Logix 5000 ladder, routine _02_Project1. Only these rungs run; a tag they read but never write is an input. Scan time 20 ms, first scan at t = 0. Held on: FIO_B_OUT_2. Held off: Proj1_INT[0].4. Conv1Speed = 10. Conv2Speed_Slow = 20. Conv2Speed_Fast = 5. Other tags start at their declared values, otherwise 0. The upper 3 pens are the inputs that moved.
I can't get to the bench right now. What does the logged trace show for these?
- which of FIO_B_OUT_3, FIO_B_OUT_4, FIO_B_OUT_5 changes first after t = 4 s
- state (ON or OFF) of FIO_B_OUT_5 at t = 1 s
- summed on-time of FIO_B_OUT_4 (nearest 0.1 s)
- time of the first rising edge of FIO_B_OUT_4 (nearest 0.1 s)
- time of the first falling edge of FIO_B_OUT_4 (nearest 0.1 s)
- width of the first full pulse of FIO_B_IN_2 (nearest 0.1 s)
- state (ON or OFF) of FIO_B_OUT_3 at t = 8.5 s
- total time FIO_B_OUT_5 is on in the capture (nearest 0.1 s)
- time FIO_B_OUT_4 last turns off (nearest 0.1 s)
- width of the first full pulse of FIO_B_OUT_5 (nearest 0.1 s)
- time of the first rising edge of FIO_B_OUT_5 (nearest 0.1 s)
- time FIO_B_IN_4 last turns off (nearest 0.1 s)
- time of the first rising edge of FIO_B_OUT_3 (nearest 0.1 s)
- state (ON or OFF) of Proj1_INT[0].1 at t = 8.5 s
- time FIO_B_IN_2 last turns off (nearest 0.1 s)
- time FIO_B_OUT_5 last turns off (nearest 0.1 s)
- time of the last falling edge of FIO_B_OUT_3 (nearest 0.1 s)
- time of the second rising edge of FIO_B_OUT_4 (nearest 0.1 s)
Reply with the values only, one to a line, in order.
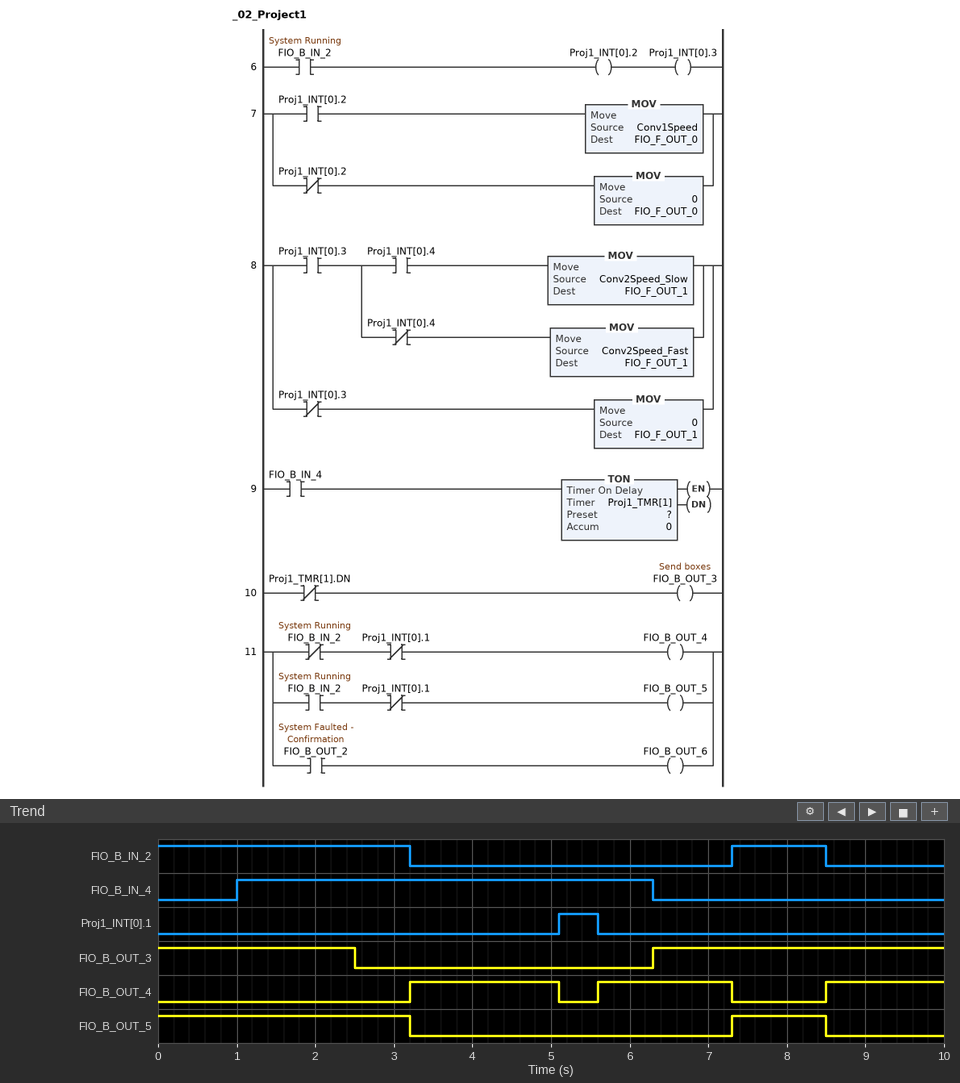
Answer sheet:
FIO_B_OUT_4
ON
5.1 s
3.2 s
5.1 s
1.2 s
ON
4.4 s
7.3 s
1.2 s
7.3 s
6.3 s
6.3 s
OFF
8.5 s
8.5 s
2.5 s
5.6 s
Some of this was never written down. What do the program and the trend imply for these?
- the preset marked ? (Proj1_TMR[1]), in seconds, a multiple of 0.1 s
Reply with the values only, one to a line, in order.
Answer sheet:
1.5 s
